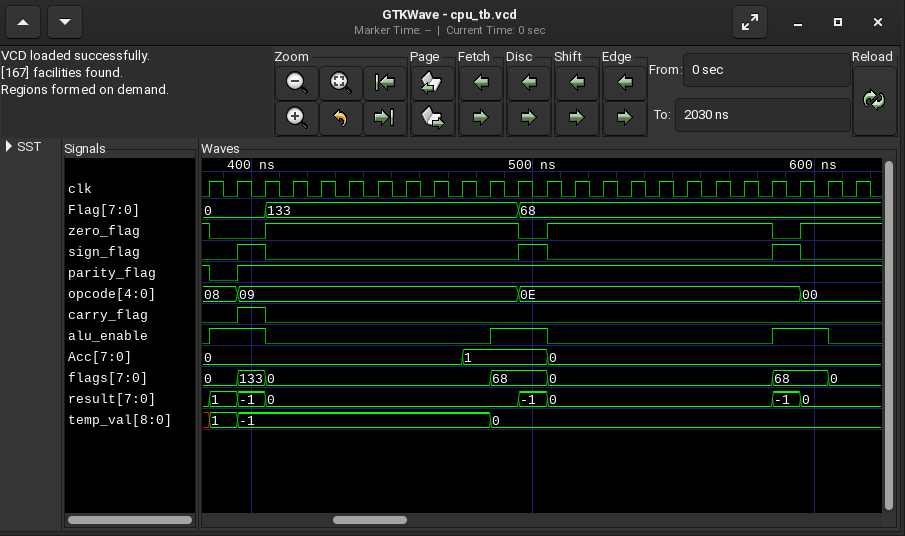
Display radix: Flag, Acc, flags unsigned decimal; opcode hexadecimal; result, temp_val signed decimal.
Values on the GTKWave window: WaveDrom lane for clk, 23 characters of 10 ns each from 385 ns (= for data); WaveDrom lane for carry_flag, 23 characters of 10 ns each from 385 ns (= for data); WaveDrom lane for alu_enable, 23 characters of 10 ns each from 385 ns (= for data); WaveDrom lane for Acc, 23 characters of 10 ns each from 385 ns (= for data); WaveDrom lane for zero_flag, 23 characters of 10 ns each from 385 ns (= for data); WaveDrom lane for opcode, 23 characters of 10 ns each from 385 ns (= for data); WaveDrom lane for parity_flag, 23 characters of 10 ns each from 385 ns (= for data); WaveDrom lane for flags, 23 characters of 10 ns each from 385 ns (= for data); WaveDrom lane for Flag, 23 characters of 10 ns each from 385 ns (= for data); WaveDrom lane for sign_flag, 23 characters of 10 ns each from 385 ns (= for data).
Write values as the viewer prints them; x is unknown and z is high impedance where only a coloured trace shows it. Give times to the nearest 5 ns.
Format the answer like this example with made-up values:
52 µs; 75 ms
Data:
{name: 'clk', wave: 'p......................'}; {name: 'carry_flag', wave: '010....................'}; {name: 'alu_enable', wave: '1.0.......1.0.......1.0'}; {name: 'Acc', wave: '=........=..=..........', data: '0 1 0'}; {name: 'zero_flag', wave: '0.1........01.......01.'}; {name: 'opcode', wave: '==.........=.........=.', data: '08 09 0E 00'}; {name: 'parity_flag', wave: '01.....................'}; {name: 'flags', wave: '===.......=.=.......=.=', data: '0 133 0 68 0 68 0'}; {name: 'Flag', wave: '=.=........=...........', data: '0 133 68'}; {name: 'sign_flag', wave: '010........10.......10.'}
